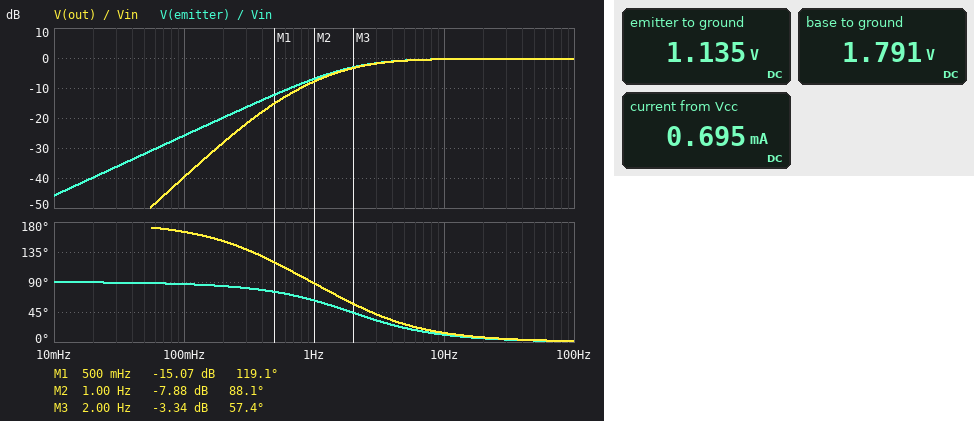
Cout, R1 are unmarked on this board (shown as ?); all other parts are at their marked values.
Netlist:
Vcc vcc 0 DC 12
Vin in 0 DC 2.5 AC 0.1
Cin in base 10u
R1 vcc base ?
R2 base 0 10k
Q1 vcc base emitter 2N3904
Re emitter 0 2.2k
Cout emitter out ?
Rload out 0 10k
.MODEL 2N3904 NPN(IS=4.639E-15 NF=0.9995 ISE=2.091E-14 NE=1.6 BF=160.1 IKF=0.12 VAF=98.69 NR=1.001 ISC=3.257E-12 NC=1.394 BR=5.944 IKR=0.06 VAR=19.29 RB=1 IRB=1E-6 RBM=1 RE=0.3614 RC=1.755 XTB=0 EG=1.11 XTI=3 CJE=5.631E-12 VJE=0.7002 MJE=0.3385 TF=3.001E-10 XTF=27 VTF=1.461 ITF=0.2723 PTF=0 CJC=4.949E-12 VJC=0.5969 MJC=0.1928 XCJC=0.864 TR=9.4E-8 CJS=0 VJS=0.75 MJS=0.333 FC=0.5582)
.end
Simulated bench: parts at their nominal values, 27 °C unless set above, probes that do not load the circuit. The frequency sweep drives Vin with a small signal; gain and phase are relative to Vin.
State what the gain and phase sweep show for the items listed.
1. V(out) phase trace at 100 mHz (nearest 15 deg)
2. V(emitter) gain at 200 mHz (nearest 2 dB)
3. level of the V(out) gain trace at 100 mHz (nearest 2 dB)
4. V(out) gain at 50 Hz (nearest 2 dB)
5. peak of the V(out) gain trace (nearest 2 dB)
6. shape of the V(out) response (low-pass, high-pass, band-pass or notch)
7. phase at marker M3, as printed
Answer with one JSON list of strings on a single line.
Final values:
["165 deg", "-20 dB", "-40 dB", "0 dB", "0 dB", "high-pass", "57.4 deg"]
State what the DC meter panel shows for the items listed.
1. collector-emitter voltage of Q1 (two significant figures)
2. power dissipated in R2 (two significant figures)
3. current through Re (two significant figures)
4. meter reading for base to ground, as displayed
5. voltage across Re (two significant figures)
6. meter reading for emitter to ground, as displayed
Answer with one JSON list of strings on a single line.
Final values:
["11 V", "320 µW", "520 µA", "1.791 V", "1.1 V", "1.135 V"]
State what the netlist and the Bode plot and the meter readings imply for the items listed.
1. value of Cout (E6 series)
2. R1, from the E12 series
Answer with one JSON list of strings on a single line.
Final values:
["33 µF", "56 kΩ"]
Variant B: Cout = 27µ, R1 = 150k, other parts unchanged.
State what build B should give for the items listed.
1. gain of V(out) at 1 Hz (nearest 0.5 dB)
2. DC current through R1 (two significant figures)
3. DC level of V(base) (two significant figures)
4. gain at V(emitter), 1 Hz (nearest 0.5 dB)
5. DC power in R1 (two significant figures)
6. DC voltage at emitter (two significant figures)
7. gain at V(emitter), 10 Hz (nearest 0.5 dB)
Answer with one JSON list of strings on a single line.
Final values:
["-9.0 dB", "75 µA", "750 mV", "-7.5 dB", "840 µW", "140 mV", "-2.0 dB"]
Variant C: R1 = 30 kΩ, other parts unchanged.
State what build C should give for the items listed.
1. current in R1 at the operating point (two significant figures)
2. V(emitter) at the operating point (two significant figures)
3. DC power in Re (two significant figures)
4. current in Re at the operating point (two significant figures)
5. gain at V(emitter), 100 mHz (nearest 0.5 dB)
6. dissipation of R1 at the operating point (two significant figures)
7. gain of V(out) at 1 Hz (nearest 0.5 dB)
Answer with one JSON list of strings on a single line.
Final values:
["300 µA", "2.3 V", "2.4 mW", "1.0 mA", "-27.0 dB", "2.7 mW", "-8.5 dB"]
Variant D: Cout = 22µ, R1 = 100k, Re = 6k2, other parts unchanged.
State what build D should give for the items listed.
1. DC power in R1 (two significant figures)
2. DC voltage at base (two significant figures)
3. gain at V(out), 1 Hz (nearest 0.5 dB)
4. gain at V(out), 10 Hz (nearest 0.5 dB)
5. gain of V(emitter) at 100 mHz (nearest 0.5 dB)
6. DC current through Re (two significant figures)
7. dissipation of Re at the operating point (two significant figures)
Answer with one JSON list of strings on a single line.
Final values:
["1.2 mW", "1.1 V", "-8.5 dB", "-1.0 dB", "-25.5 dB", "77 µA", "37 µW"]
